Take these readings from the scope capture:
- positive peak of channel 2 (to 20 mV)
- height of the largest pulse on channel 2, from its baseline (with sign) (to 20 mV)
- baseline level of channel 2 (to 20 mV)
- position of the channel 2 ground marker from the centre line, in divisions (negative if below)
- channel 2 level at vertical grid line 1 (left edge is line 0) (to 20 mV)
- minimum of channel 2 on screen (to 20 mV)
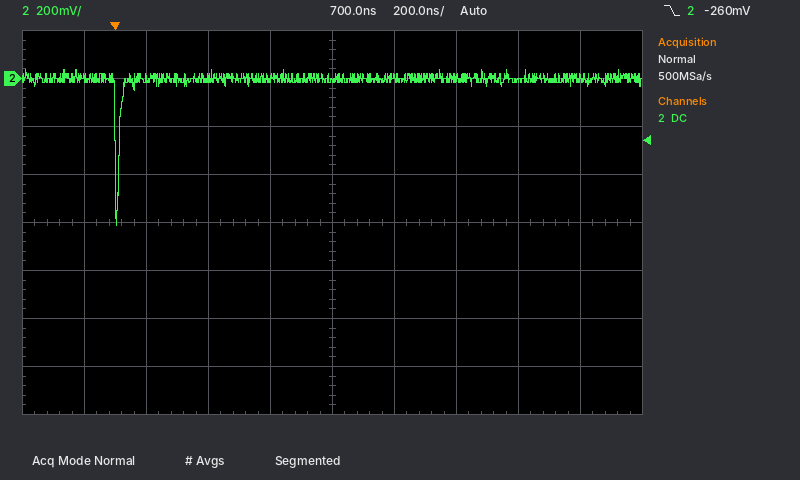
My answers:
40 mV
-620 mV
0 mV
+3.0 div
0 mV
-620 mV
